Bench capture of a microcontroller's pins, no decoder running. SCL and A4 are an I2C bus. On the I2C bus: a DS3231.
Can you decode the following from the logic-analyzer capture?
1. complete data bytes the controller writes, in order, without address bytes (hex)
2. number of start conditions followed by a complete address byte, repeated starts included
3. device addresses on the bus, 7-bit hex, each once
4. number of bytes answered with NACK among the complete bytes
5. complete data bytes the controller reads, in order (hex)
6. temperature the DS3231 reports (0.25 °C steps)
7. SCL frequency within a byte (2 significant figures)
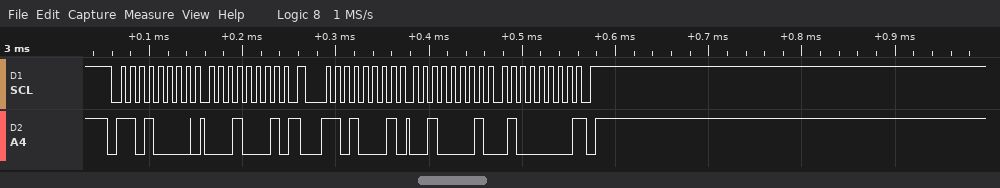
11
2
0x68
1
21 40
33.25 °C
100 kHz
